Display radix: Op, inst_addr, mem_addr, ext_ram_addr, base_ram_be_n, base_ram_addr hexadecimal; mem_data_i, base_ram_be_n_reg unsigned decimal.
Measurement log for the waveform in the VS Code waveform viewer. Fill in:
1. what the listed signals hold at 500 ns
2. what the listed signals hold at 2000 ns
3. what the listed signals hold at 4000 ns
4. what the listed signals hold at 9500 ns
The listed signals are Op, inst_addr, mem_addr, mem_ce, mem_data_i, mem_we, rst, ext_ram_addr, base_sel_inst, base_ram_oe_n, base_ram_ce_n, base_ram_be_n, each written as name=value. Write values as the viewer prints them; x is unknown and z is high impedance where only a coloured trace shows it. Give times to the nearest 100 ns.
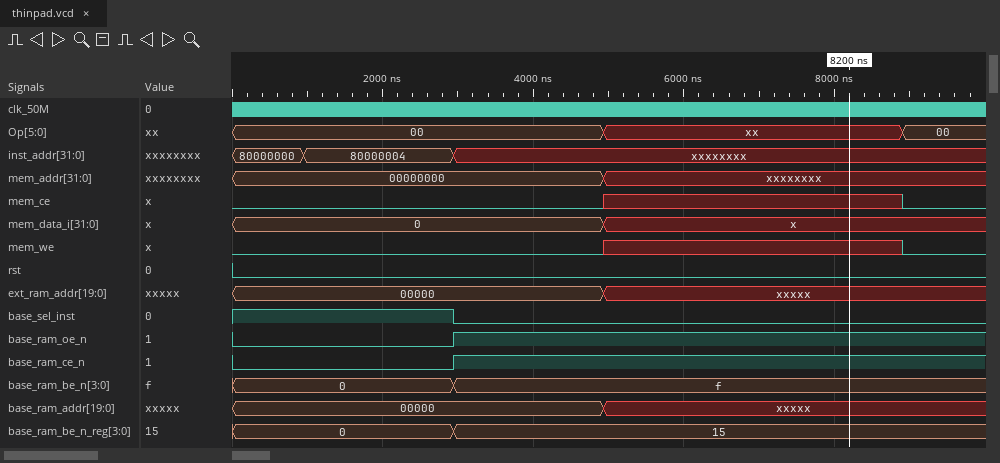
Op=00, inst_addr=80000000, mem_addr=00000000, mem_ce=0, mem_data_i=0, mem_we=0, rst=0, ext_ram_addr=00000, base_sel_inst=1, base_ram_oe_n=0, base_ram_ce_n=0, base_ram_be_n=0
Op=00, inst_addr=80000004, mem_addr=00000000, mem_ce=0, mem_data_i=0, mem_we=0, rst=0, ext_ram_addr=00000, base_sel_inst=1, base_ram_oe_n=0, base_ram_ce_n=0, base_ram_be_n=0
Op=00, inst_addr=xxxxxxxx, mem_addr=00000000, mem_ce=0, mem_data_i=0, mem_we=0, rst=0, ext_ram_addr=00000, base_sel_inst=0, base_ram_oe_n=1, base_ram_ce_n=1, base_ram_be_n=f
Op=00, inst_addr=xxxxxxxx, mem_addr=xxxxxxxx, mem_ce=0, mem_data_i=x, mem_we=0, rst=0, ext_ram_addr=xxxxx, base_sel_inst=0, base_ram_oe_n=1, base_ram_ce_n=1, base_ram_be_n=f
